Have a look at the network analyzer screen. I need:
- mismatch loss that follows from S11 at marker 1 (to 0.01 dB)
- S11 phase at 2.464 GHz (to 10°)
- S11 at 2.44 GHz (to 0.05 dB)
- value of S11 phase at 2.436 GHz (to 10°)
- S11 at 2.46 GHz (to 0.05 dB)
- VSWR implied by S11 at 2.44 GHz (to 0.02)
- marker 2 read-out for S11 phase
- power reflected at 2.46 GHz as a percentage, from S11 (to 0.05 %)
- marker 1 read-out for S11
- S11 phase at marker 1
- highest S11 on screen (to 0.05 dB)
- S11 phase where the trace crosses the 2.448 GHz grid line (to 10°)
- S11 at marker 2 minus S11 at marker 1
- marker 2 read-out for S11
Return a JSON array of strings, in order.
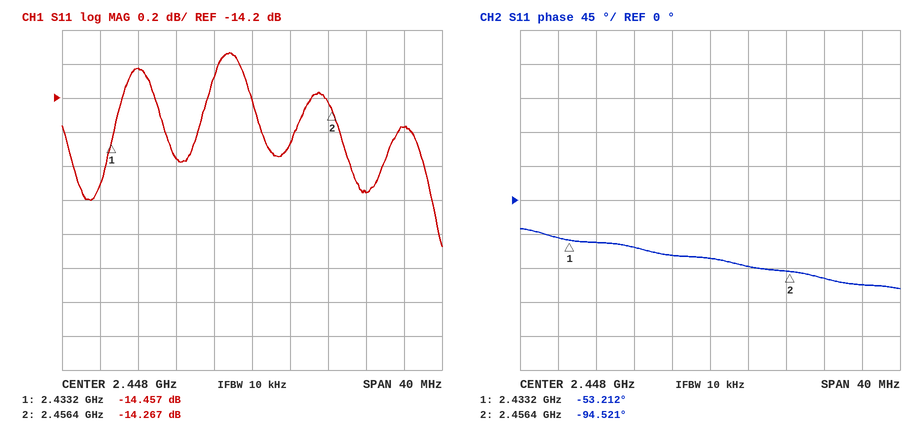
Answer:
["0.16 dB", "-110°", "-14.55 dB", "-60°", "-14.75 dB", "1.46", "-94.521°", "3.35 %", "-14.457 dB", "-53.212°", "-13.95 dB", "-80°", "0.190 dB", "-14.267 dB"]
